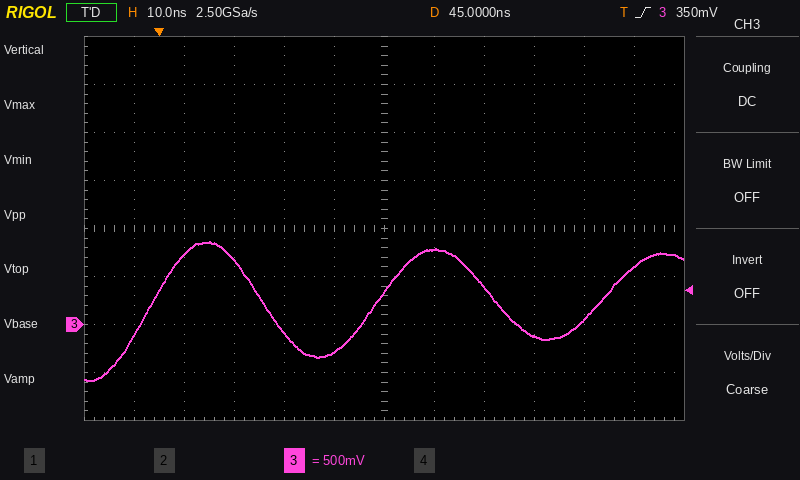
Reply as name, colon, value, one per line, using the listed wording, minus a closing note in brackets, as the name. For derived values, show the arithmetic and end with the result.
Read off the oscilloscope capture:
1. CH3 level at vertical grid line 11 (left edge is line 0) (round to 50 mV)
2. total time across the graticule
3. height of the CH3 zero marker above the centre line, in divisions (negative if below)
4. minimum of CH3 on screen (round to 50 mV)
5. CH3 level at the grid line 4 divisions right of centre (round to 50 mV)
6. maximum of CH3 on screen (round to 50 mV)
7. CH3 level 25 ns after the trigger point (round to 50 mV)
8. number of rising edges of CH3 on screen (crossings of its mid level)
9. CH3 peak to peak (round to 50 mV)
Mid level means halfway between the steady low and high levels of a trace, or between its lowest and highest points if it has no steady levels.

CH3 level at vertical grid line 11 (left edge is line 0): 600 mV
total time across the graticule: 120 ns
height of the CH3 zero marker above the centre line, in divisions: -2.0 div
minimum of CH3 on screen: -600 mV
CH3 level at the grid line 4 divisions right of centre: 50 mV
maximum of CH3 on screen: 850 mV
CH3 level 25 ns after the trigger point: -100 mV
number of rising edges of CH3 on screen: 3
CH3 peak to peak: 850 mV − (-600 mV) = 1.45 V
